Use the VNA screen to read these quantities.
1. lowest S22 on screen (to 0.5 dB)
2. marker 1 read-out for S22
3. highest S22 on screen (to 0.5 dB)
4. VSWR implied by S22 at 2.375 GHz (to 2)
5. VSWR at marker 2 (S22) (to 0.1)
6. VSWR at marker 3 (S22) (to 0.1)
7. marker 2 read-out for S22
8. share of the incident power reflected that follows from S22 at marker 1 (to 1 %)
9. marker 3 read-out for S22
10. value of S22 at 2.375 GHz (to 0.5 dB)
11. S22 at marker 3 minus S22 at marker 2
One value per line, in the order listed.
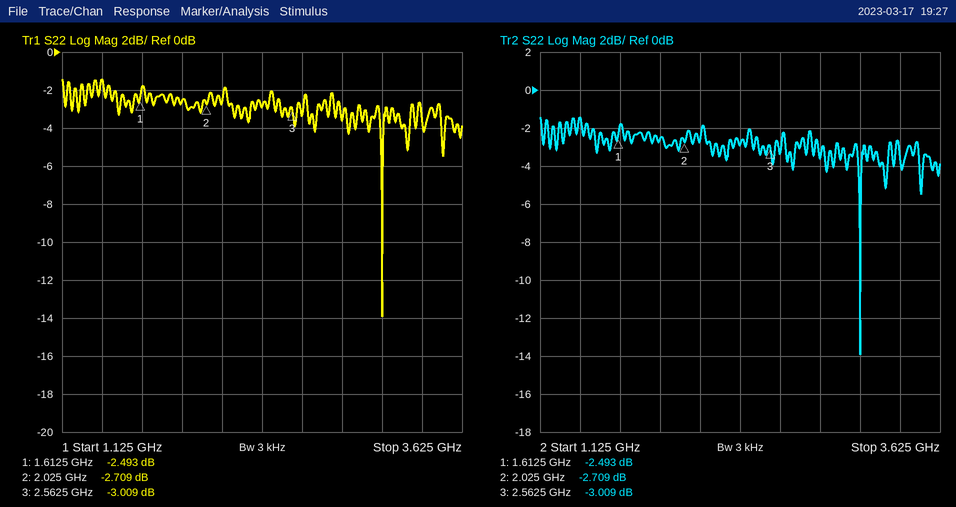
-14.0 dB
-2.493 dB
-1.5 dB
6
6.5
5.8
-2.709 dB
56 %
-3.009 dB
-3.0 dB
-0.300 dB
